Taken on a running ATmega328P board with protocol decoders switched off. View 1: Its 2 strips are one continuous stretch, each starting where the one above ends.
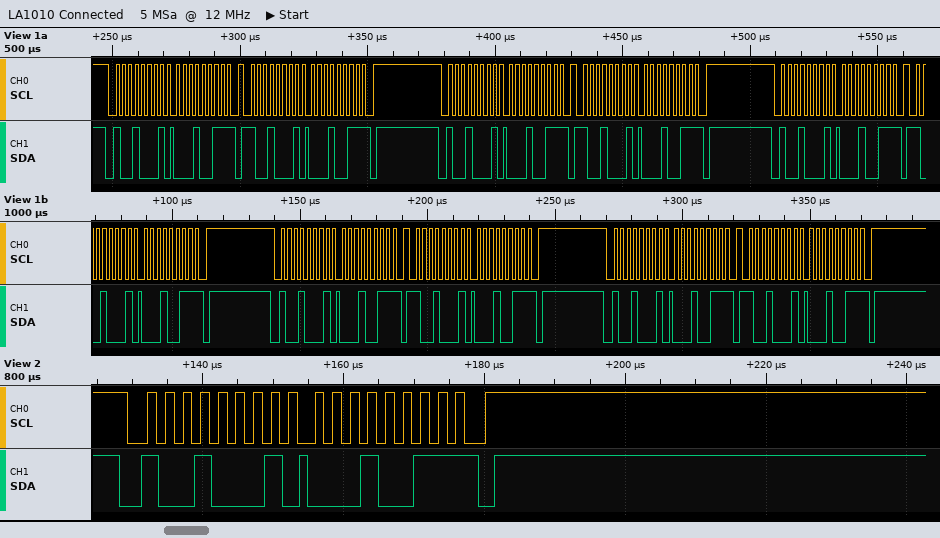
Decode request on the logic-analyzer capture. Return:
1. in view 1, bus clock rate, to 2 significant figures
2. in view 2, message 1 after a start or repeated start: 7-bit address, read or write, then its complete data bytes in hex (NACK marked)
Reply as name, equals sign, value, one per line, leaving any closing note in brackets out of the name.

in view 1, bus clock rate, to 2 significant figures = 400 kHz
in view 2, message 1 after a start or repeated start: 7-bit address, read or write, then its complete data bytes in hex = 0x48 read: 13 NACK
